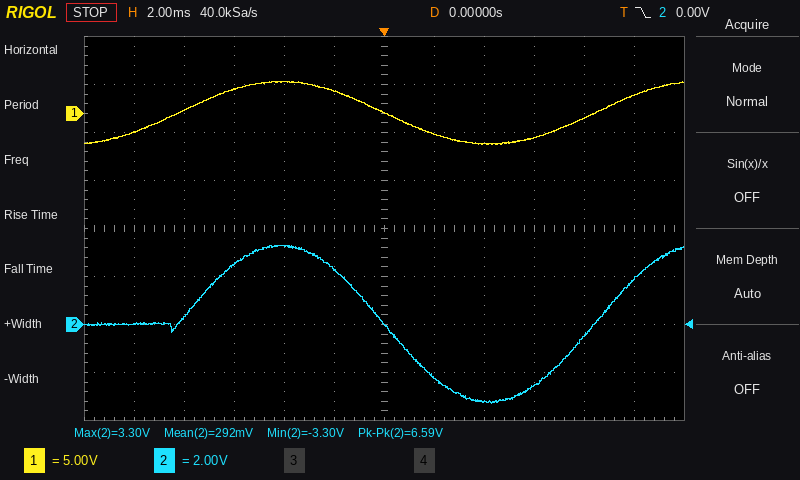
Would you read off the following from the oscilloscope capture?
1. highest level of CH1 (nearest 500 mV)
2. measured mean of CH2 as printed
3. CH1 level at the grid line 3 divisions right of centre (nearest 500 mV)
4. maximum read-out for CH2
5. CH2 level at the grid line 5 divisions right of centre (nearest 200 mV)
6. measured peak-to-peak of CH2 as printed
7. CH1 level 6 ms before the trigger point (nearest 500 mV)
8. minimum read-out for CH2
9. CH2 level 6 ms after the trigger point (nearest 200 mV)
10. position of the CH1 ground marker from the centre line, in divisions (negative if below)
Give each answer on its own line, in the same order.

3.5 V
292 mV
-2.5 V
3.30 V
1.8 V
6.59 V
2.5 V
-3.30 V
-2.6 V
+2.4 div
